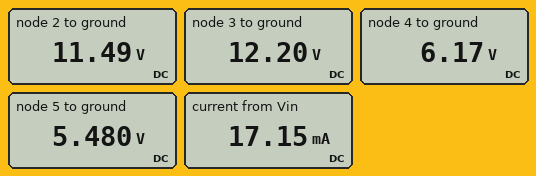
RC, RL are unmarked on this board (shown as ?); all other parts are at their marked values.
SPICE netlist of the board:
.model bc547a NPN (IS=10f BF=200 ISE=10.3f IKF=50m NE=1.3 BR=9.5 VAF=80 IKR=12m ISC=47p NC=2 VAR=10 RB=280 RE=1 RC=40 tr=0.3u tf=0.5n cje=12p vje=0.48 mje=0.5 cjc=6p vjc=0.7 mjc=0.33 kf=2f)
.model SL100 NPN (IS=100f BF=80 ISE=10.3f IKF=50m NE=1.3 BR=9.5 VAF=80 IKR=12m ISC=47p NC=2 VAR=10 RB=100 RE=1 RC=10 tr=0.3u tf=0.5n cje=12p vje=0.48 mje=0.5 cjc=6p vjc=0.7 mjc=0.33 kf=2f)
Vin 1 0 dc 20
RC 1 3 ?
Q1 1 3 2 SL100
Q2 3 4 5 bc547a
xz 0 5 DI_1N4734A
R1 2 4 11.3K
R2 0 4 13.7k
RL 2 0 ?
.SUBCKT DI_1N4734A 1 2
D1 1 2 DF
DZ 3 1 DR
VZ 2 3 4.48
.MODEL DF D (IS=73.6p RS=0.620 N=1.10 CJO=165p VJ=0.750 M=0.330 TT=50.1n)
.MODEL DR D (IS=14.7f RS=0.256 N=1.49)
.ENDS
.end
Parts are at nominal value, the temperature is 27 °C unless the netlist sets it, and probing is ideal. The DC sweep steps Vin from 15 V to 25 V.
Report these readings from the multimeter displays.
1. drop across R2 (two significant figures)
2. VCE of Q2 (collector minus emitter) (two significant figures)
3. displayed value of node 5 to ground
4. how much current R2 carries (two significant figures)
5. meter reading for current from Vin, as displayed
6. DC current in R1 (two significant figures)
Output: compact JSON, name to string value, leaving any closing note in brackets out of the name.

{"drop across R2": "6.2 V", "VCE of Q2 (collector minus emitter)": "6.7 V", "displayed value of node 5 to ground": "5.480 V", "how much current R2 carries": "450 µA", "meter reading for current from Vin, as displayed": "17.15 mA", "DC current in R1": "470 µA"}
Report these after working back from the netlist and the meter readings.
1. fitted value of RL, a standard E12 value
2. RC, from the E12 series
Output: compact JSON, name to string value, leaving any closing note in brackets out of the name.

{"fitted value of RL, a standard E12 value": "820 Ω", "RC, from the E12 series": "2.7 kΩ"}
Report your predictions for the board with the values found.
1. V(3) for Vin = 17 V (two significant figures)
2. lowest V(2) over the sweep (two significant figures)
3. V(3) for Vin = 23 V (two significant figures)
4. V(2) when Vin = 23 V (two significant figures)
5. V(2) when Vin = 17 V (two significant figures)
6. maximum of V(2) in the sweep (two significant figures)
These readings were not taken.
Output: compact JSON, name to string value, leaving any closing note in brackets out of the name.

{"V(3) for Vin = 17 V": "12 V", "lowest V(2) over the sweep": "11 V", "V(3) for Vin = 23 V": "12 V", "V(2) when Vin = 23 V": "12 V", "V(2) when Vin = 17 V": "11 V", "maximum of V(2) in the sweep": "12 V"}
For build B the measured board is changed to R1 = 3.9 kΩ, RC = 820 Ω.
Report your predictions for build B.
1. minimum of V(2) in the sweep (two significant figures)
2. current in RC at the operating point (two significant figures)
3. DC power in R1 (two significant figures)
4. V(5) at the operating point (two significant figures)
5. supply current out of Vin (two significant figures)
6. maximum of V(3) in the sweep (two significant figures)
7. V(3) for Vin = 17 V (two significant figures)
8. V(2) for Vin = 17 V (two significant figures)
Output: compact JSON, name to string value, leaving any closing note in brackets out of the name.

{"minimum of V(2) in the sweep": "8.3 V", "current in RC at the operating point": "13 mA", "DC power in R1": "1.3 mW", "V(5) at the operating point": "5.5 V", "supply current out of Vin": "24 mA", "maximum of V(3) in the sweep": "9.5 V", "V(3) for Vin = 17 V": "9.1 V", "V(2) for Vin = 17 V": "8.4 V"}
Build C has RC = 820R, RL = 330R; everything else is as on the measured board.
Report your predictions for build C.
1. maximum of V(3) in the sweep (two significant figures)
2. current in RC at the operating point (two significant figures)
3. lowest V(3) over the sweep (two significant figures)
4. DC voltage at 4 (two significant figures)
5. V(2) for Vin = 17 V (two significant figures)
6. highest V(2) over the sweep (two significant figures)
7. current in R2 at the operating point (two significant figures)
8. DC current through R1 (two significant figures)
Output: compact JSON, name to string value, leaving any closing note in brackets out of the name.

{"maximum of V(3) in the sweep": "14 V", "current in RC at the operating point": "8.6 mA", "lowest V(3) over the sweep": "12 V", "DC voltage at 4": "6.3 V", "V(2) for Vin = 17 V": "12 V", "highest V(2) over the sweep": "13 V", "current in R2 at the operating point": "460 µA", "DC current through R1": "520 µA"}
